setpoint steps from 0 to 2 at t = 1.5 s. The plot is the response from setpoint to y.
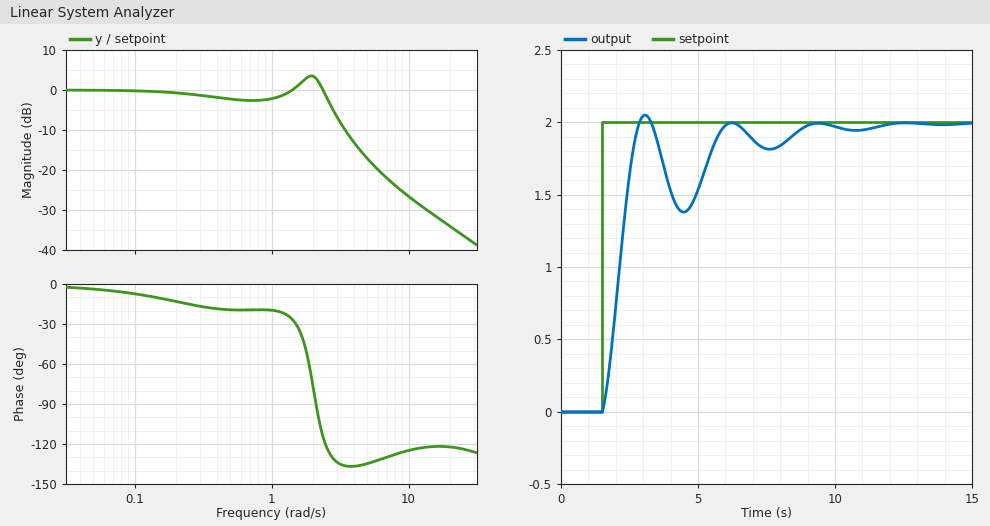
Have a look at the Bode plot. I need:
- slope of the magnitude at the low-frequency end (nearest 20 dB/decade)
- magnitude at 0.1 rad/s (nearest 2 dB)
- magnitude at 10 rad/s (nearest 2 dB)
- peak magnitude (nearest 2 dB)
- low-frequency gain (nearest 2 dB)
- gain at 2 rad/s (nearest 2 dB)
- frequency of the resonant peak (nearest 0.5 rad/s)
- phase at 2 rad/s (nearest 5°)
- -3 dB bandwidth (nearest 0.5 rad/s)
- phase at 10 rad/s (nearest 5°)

0 dB/decade
0 dB
-26 dB
4 dB
0 dB
4 dB
2.0 rad/s
-75°
2.5 rad/s
-125°
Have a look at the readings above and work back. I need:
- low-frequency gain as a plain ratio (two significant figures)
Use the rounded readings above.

1.0
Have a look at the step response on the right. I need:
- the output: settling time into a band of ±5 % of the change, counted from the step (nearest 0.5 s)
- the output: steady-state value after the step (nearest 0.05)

7.0 s
2.00
